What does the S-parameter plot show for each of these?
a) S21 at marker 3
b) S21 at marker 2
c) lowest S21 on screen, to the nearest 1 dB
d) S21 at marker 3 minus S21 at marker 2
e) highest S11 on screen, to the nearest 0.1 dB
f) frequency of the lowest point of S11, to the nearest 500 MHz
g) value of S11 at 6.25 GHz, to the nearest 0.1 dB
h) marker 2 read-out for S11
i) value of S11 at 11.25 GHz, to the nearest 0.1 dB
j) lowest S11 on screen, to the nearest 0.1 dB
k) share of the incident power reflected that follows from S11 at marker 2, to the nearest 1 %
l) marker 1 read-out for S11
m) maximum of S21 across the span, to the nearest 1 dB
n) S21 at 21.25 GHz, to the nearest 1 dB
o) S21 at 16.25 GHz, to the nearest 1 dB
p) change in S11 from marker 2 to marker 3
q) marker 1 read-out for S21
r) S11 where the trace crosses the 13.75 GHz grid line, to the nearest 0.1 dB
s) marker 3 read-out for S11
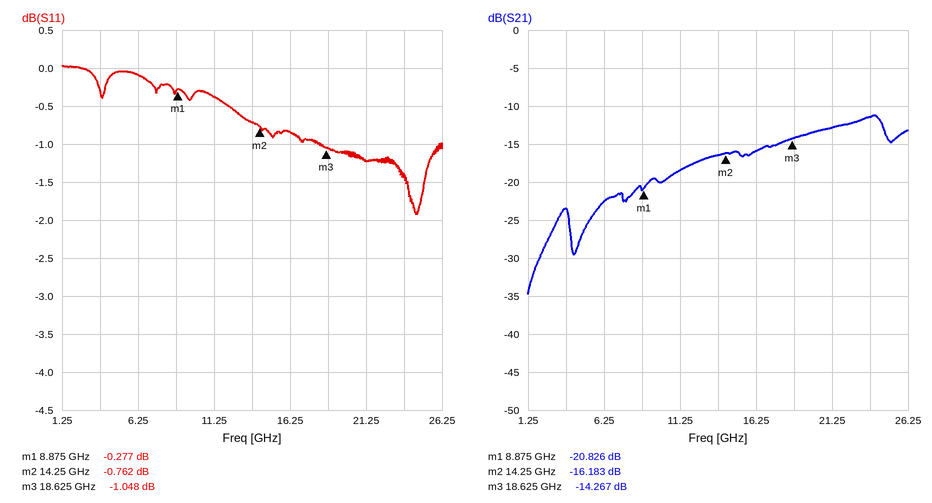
-14.267 dB
-16.183 dB
-35 dB
1.916 dB
0.0 dB
24.5 GHz
-0.1 dB
-0.762 dB
-0.4 dB
-1.9 dB
84 %
-0.277 dB
-11 dB
-13 dB
-16 dB
-0.286 dB
-20.826 dB
-0.7 dB
-1.048 dB
